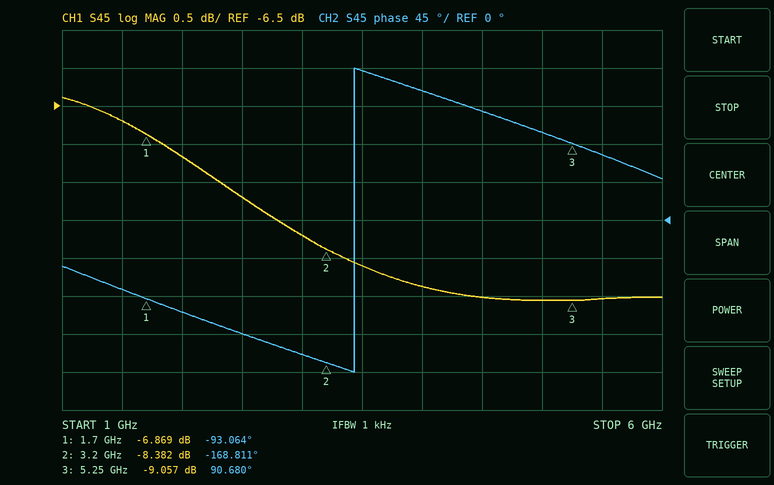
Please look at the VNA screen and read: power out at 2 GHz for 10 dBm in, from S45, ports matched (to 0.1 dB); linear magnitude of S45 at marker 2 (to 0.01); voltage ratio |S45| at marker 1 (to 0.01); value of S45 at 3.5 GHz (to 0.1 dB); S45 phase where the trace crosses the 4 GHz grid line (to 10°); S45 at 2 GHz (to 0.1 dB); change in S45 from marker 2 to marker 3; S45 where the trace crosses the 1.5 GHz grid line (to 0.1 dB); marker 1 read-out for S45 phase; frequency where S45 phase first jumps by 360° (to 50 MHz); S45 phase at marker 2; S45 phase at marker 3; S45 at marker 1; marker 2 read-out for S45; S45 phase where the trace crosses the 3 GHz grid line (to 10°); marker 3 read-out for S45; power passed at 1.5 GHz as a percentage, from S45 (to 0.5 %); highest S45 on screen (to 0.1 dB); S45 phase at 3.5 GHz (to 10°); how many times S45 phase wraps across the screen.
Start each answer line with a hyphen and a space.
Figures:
- 2.8 dBm
- 0.38
- 0.45
- -8.6 dB
- 150°
- -7.2 dB
- -0.675 dB
- -6.7 dB
- -93.064°
- 3.45 GHz
- -168.811°
- 90.680°
- -6.869 dB
- -8.382 dB
- -160°
- -9.057 dB
- 21.5 %
- -6.4 dB
- 180°
- 1
